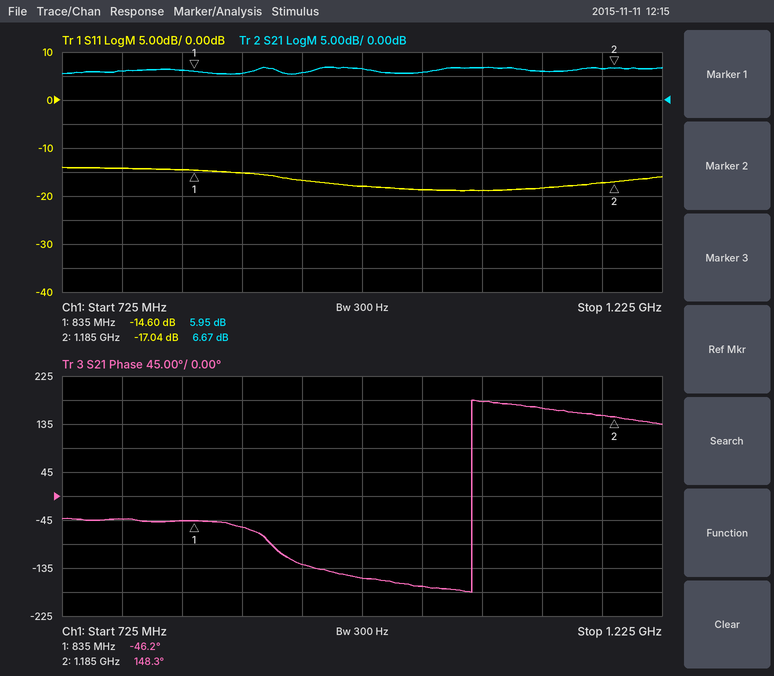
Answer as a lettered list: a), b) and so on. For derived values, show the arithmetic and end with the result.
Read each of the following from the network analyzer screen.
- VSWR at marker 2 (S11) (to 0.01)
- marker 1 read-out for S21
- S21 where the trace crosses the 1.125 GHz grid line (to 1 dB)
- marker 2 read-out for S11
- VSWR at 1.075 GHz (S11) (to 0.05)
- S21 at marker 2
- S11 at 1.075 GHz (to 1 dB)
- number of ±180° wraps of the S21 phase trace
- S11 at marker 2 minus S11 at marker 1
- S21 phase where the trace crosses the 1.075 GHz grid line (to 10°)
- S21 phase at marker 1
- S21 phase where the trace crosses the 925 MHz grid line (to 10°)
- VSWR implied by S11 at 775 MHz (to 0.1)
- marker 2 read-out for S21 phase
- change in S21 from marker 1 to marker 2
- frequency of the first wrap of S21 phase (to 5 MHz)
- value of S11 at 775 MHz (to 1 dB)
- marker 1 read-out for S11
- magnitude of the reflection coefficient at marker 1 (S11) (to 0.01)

a) (1 + 0.1406)/(1 − 0.1406) ≈ 1.33
b) 5.95 dB
c) 6 dB
d) -17.04 dB
e) |Γ| = 10^(-19/20) = 0.1122; VSWR = (1 + 0.1122)/(1 − 0.1122) ≈ 1.25
f) 6.67 dB
g) -19 dB
h) 1
i) -17.04 − (-14.6) = -2.44 dB
j) 180°
k) -46.2°
l) -130°
m) |Γ| = 10^(-14/20) = 0.1995; VSWR = (1 + 0.1995)/(1 − 0.1995) ≈ 1.5
n) 148.3°
o) 6.67 − (5.95) = 0.72 dB
p) 1.065 GHz
q) -14 dB
r) -14.60 dB
s) 10^(-14.6/20) ≈ 0.19
